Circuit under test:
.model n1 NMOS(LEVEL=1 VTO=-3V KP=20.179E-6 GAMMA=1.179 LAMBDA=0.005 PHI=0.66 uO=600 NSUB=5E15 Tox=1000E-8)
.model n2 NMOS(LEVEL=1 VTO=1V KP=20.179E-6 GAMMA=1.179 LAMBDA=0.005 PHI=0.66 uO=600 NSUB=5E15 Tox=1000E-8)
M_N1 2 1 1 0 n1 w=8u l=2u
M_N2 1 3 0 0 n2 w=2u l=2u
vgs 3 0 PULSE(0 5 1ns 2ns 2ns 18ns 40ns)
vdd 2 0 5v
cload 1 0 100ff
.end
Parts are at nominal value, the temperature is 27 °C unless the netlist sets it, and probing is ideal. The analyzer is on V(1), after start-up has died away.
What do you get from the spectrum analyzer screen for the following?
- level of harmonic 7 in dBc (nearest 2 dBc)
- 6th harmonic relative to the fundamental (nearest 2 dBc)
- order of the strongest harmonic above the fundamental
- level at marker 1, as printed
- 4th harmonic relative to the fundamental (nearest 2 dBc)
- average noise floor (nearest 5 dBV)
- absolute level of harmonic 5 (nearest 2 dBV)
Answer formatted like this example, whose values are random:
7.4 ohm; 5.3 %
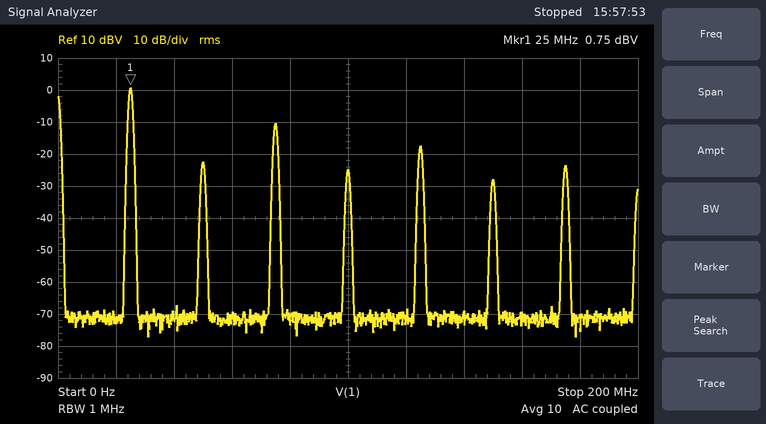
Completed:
-24 dBc; -28 dBc; 3; 0.75 dBV; -26 dBc; -70 dBV; -18 dBV
